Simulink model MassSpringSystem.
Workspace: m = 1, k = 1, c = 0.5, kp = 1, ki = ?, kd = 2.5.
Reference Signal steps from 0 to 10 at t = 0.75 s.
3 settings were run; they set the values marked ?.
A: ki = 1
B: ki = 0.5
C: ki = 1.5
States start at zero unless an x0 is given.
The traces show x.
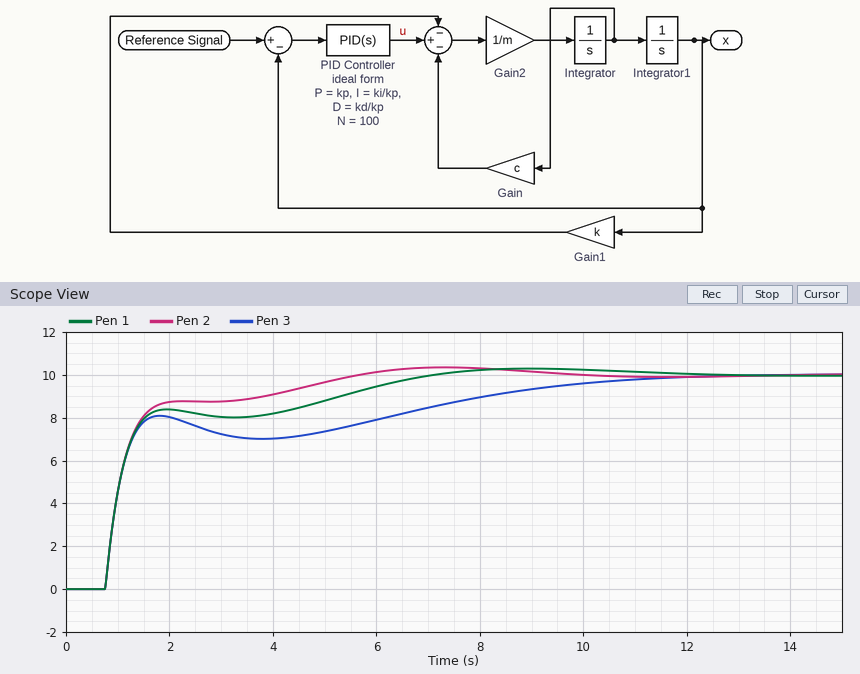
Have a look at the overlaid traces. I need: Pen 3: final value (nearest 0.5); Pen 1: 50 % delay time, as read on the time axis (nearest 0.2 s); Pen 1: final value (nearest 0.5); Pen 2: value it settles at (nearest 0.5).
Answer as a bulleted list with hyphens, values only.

- 10.0
- 1.0 s
- 10.0
- 10.0
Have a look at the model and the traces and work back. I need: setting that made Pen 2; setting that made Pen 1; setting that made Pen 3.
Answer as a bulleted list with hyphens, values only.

- C
- A
- B
